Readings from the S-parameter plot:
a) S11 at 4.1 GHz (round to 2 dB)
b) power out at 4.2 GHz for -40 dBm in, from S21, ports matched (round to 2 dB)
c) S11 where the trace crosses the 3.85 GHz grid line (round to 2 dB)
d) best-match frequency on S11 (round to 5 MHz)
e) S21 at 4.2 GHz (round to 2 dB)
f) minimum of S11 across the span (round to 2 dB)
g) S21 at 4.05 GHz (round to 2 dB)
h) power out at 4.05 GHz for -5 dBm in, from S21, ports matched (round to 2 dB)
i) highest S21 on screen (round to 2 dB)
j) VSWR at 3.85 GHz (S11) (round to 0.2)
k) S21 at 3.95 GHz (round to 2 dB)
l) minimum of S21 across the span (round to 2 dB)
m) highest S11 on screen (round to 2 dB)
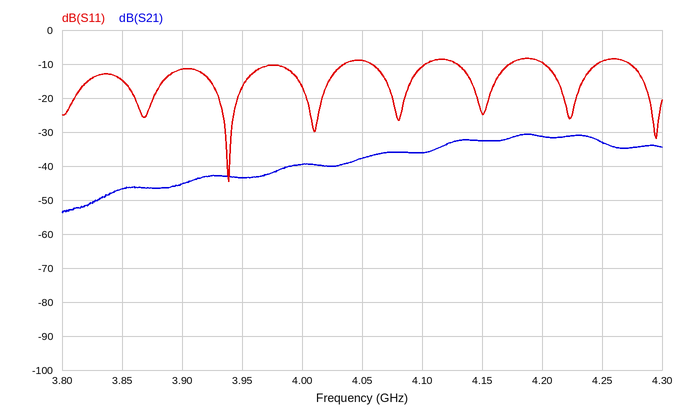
-10 dB
-72 dBm
-14 dB
3.940 GHz
-32 dB
-44 dB
-38 dB
-42 dBm
-30 dB
1.4
-44 dB
-54 dB
-8 dB
